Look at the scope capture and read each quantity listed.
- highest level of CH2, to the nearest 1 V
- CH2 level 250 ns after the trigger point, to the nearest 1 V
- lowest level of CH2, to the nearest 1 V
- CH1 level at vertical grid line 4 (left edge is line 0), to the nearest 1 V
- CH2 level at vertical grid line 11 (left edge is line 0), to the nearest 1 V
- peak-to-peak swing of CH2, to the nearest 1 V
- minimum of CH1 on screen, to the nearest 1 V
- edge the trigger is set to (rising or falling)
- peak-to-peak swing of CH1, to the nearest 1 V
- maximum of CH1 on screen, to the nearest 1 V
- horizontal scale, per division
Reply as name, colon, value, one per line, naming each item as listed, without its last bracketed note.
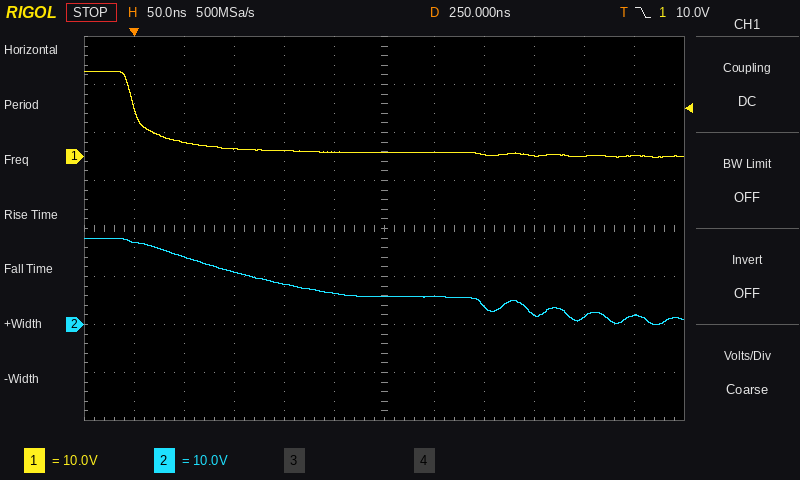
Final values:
highest level of CH2, to the nearest 1 V: 18 V
CH2 level 250 ns after the trigger point, to the nearest 1 V: 6 V
lowest level of CH2, to the nearest 1 V: 0 V
CH1 level at vertical grid line 4 (left edge is line 0), to the nearest 1 V: 1 V
CH2 level at vertical grid line 11 (left edge is line 0), to the nearest 1 V: 2 V
peak-to-peak swing of CH2, to the nearest 1 V: 18 V
minimum of CH1 on screen, to the nearest 1 V: 0 V
edge the trigger is set to: falling
peak-to-peak swing of CH1, to the nearest 1 V: 18 V
maximum of CH1 on screen, to the nearest 1 V: 18 V
horizontal scale, per division: 50 ns
